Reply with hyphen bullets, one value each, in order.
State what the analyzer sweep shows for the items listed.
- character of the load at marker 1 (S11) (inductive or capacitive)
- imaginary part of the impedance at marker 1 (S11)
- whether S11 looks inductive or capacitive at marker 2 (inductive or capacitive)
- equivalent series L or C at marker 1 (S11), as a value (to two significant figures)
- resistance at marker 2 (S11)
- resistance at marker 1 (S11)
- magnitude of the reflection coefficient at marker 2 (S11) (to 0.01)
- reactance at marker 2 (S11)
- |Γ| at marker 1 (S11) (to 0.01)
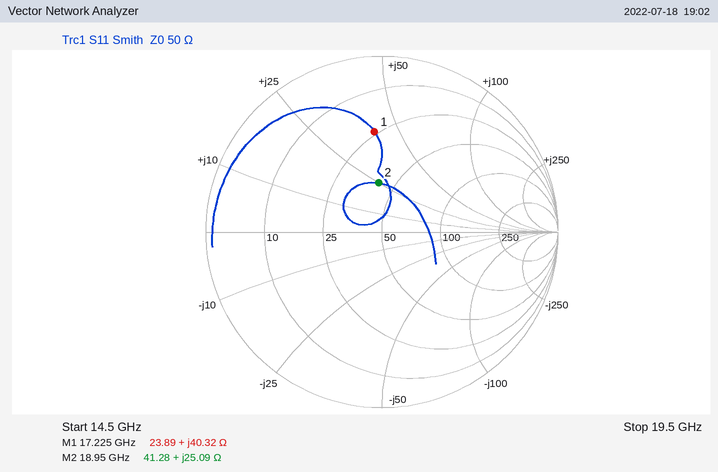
- inductive
- +40.32 Ω
- inductive
- 370 pH
- 41.28 Ω
- 23.89 Ω
- 0.28
- +25.09 Ω
- 0.57
